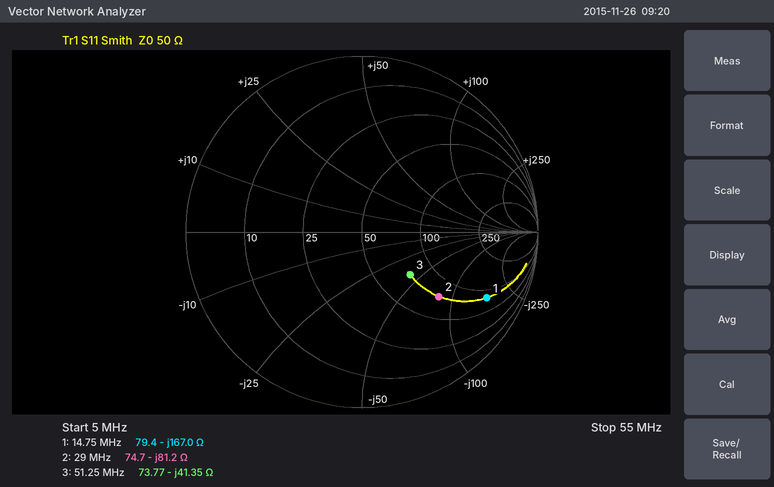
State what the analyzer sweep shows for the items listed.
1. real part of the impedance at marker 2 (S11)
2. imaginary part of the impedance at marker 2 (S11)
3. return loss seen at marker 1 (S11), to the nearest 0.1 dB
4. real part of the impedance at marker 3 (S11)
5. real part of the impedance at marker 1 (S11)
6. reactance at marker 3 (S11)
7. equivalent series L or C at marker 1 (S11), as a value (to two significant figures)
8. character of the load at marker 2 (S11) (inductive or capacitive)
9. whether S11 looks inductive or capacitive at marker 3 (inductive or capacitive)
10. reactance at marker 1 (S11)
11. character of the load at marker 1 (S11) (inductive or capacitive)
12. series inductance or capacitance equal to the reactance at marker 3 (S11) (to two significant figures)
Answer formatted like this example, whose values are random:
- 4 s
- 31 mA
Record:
- 74.7 Ω
- -81.2 Ω
- 1.9 dB
- 73.77 Ω
- 79.4 Ω
- -41.35 Ω
- 65 pF
- capacitive
- capacitive
- -167.0 Ω
- capacitive
- 75 pF
